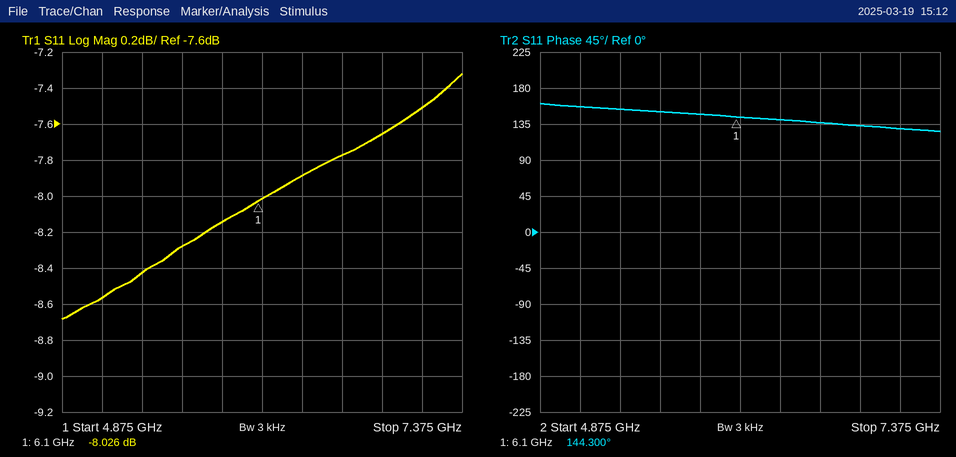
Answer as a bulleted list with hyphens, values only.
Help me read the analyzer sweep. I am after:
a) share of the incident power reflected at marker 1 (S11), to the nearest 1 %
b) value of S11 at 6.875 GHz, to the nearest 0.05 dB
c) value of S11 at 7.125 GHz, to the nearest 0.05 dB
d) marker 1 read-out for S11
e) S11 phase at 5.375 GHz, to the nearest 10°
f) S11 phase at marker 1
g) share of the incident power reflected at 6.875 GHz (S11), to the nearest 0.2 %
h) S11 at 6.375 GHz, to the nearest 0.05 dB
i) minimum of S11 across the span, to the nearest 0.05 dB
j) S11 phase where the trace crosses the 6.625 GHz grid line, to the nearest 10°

- 16 %
- -7.65 dB
- -7.50 dB
- -8.026 dB
- 150°
- 144.300°
- 17.2 %
- -7.90 dB
- -8.70 dB
- 140°
